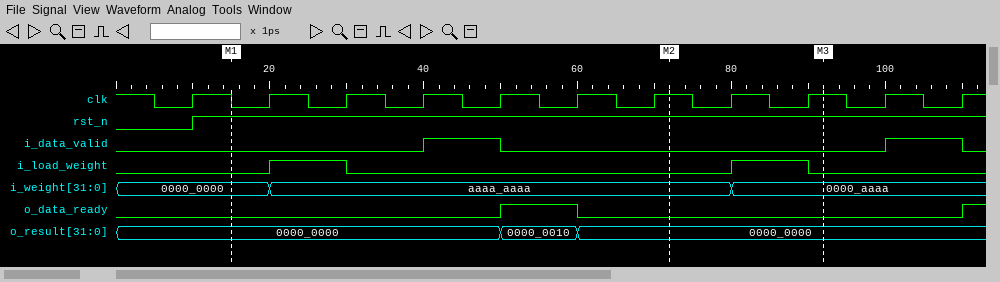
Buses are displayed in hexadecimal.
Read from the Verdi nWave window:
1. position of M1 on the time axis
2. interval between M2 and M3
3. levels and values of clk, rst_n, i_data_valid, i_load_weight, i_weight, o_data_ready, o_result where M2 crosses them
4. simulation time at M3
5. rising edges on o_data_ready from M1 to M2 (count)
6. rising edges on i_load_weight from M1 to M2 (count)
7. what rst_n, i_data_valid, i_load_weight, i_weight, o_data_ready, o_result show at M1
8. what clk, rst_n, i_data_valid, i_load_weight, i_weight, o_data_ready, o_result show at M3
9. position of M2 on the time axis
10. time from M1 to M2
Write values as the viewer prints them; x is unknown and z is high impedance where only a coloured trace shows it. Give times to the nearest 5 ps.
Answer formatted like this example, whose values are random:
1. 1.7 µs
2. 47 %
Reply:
1. 15 ps
2. 20 ps
3. clk=1, rst_n=1, i_data_valid=0, i_load_weight=0, i_weight=aaaa_aaaa, o_data_ready=0, o_result=0000_0000
4. 90 ps
5. 1
6. 1
7. rst_n=1, i_data_valid=0, i_load_weight=0, i_weight=0000_0000, o_data_ready=0, o_result=0000_0000
8. clk=1, rst_n=1, i_data_valid=0, i_load_weight=0, i_weight=0000_aaaa, o_data_ready=0, o_result=0000_0000
9. 70 ps
10. 55 ps
